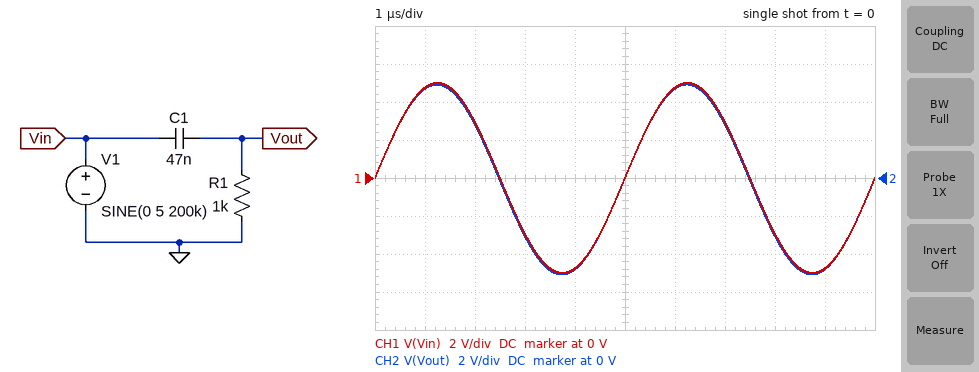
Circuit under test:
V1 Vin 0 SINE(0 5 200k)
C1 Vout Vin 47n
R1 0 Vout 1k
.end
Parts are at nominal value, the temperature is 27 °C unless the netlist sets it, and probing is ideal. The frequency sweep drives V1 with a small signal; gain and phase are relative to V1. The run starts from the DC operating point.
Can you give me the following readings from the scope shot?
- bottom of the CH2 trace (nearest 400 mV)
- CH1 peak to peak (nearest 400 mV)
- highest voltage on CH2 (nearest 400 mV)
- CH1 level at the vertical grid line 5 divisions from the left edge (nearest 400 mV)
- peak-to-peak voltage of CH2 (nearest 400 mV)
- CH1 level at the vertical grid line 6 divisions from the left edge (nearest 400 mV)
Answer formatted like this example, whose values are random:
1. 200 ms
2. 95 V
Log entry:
1. -5.2 V
2. 10.0 V
3. 4.8 V
4. 0 V
5. 10.0 V
6. 4.8 V
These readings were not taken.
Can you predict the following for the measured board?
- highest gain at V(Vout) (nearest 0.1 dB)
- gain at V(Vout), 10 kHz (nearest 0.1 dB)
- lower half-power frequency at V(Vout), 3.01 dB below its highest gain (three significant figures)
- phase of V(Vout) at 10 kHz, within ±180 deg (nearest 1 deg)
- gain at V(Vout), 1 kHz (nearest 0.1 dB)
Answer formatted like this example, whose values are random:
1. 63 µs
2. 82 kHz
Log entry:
1. 0 dB
2. -0.5 dB
3. 3.39 kHz
4. 19 deg
5. -11.0 dB
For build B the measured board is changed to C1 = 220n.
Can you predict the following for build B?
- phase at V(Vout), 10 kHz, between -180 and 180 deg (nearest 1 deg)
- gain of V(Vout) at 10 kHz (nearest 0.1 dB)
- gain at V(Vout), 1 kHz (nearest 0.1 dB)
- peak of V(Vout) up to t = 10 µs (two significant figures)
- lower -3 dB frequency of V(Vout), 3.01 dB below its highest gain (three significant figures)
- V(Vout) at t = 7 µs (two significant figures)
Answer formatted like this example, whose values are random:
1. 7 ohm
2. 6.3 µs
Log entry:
1. 4 deg
2. 0 dB
3. -1.8 dB
4. 5.0 V
5. 723 Hz
6. 2.9 V
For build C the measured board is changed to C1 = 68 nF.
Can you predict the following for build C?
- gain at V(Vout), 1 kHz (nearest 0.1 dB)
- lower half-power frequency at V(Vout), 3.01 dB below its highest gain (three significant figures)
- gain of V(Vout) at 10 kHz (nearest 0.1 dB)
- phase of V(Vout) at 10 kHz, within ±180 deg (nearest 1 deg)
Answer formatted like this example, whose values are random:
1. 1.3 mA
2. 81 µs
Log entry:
1. -8.1 dB
2. 2.34 kHz
3. -0.2 dB
4. 13 deg
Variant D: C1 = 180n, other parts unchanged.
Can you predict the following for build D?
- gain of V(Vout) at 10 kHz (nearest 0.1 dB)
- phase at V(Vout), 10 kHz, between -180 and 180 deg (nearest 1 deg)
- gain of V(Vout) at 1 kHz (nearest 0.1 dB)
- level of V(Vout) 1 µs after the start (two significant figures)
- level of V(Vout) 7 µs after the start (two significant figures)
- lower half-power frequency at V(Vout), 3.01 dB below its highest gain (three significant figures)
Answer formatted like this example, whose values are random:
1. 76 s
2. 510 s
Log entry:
1. 0 dB
2. 5 deg
3. -2.5 dB
4. 4.7 V
5. 2.9 V
6. 884 Hz
